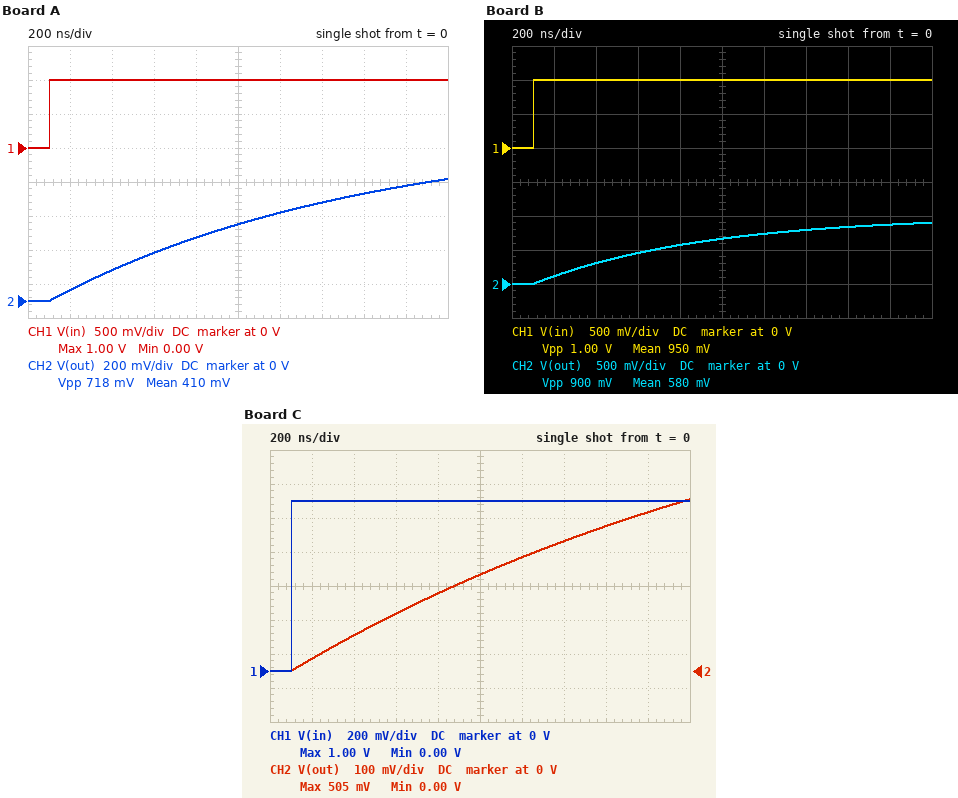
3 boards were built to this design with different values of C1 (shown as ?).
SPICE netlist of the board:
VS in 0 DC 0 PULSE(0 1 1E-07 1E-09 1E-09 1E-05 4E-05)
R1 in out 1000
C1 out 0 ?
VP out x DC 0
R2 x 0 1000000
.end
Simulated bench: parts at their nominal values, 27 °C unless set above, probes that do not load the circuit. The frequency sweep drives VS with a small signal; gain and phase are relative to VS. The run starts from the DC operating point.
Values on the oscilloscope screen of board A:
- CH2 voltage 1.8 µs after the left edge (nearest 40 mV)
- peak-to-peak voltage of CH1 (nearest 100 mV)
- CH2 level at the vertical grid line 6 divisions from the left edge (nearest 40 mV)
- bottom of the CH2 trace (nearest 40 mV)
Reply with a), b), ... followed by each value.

a) 680 mV
b) 1.0 V
c) 520 mV
d) 0 V
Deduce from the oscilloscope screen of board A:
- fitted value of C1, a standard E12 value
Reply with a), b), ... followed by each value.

a) 1.5 nF
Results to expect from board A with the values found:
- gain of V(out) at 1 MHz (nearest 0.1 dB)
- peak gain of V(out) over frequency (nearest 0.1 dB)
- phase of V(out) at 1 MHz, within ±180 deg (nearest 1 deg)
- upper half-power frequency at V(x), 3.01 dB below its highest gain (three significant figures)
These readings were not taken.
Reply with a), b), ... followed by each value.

a) -19.5 dB
b) 0 dB
c) -84 deg
d) 106 kHz
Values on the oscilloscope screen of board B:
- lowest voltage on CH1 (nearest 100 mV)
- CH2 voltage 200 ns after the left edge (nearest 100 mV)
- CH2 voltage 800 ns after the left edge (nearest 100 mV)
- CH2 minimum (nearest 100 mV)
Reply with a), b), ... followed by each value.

a) 0 V
b) 100 mV
c) 600 mV
d) 0 V
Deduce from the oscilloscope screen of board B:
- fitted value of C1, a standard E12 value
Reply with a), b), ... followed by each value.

a) 820 pF
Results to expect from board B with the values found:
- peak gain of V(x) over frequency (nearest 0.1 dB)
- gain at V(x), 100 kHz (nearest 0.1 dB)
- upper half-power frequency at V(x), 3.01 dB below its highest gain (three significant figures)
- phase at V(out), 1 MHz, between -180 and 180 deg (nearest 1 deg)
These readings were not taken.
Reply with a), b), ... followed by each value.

a) 0 dB
b) -1.0 dB
c) 194 kHz
d) -79 deg
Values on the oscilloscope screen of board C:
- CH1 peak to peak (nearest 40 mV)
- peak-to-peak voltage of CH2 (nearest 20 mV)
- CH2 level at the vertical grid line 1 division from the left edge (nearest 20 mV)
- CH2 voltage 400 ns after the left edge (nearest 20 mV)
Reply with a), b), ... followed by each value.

a) 1.00 V
b) 500 mV
c) 40 mV
d) 100 mV
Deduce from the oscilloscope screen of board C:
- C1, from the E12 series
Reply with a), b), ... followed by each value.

a) 2.7 nF
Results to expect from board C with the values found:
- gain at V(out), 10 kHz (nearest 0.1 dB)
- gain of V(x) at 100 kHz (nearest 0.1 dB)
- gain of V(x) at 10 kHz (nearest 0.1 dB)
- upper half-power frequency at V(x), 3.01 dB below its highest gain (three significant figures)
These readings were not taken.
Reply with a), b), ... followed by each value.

a) -0.1 dB
b) -5.9 dB
c) -0.1 dB
d) 59.0 kHz
